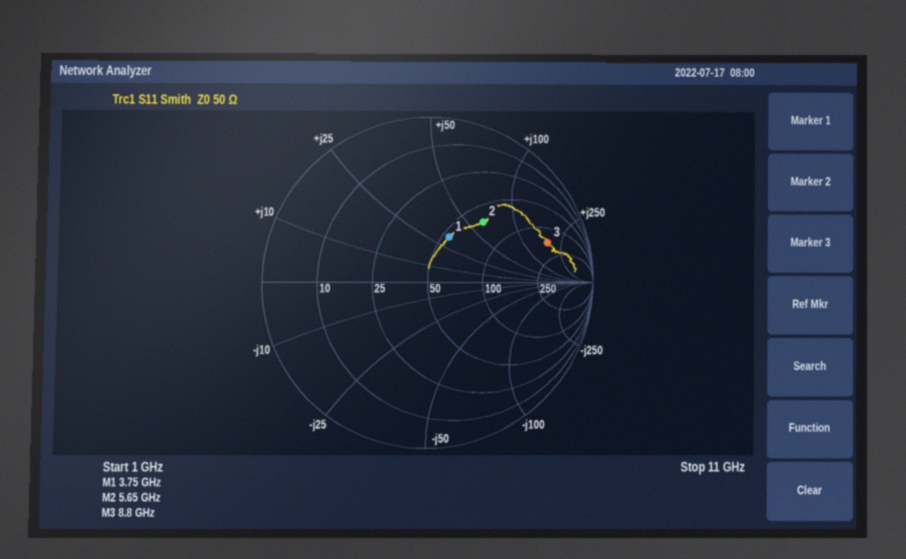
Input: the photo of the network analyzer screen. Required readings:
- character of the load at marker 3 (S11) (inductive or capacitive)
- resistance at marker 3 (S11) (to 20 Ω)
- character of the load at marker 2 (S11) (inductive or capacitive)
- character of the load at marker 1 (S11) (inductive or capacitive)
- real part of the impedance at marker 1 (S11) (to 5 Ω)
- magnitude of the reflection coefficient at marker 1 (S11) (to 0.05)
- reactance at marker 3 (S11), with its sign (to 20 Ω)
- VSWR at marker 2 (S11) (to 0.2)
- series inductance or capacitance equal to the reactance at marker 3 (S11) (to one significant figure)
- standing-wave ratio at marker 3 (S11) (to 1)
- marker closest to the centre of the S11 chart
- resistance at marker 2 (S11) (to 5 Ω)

inductive
160 Ω
inductive
inductive
55 Ω
0.30
+180 Ω
3.0
3 nH
7
marker 1
65 Ω
